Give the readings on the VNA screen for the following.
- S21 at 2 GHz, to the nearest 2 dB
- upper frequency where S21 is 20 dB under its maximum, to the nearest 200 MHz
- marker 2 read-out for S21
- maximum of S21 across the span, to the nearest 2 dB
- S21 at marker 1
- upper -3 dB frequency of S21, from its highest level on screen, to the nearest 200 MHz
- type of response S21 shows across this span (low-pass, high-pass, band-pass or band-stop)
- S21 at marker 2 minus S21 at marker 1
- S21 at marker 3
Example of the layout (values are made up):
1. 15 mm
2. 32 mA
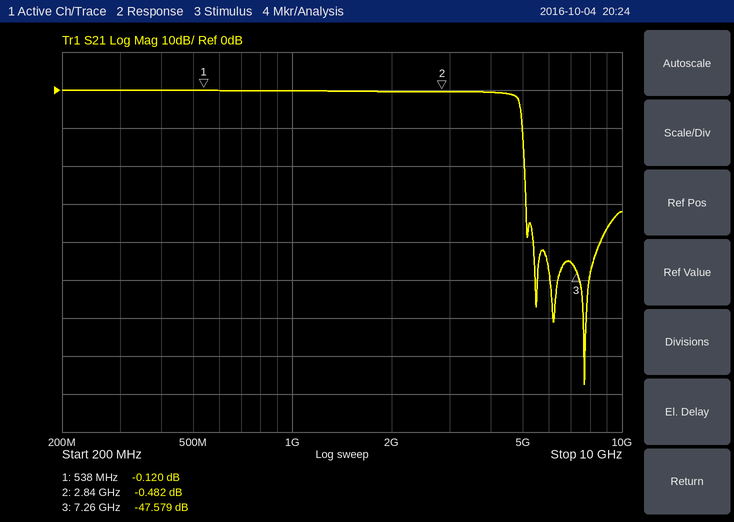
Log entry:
1. 0 dB
2. 5.0 GHz
3. -0.482 dB
4. 0 dB
5. -0.120 dB
6. 4.8 GHz
7. low-pass
8. -0.362 dB
9. -47.579 dB
